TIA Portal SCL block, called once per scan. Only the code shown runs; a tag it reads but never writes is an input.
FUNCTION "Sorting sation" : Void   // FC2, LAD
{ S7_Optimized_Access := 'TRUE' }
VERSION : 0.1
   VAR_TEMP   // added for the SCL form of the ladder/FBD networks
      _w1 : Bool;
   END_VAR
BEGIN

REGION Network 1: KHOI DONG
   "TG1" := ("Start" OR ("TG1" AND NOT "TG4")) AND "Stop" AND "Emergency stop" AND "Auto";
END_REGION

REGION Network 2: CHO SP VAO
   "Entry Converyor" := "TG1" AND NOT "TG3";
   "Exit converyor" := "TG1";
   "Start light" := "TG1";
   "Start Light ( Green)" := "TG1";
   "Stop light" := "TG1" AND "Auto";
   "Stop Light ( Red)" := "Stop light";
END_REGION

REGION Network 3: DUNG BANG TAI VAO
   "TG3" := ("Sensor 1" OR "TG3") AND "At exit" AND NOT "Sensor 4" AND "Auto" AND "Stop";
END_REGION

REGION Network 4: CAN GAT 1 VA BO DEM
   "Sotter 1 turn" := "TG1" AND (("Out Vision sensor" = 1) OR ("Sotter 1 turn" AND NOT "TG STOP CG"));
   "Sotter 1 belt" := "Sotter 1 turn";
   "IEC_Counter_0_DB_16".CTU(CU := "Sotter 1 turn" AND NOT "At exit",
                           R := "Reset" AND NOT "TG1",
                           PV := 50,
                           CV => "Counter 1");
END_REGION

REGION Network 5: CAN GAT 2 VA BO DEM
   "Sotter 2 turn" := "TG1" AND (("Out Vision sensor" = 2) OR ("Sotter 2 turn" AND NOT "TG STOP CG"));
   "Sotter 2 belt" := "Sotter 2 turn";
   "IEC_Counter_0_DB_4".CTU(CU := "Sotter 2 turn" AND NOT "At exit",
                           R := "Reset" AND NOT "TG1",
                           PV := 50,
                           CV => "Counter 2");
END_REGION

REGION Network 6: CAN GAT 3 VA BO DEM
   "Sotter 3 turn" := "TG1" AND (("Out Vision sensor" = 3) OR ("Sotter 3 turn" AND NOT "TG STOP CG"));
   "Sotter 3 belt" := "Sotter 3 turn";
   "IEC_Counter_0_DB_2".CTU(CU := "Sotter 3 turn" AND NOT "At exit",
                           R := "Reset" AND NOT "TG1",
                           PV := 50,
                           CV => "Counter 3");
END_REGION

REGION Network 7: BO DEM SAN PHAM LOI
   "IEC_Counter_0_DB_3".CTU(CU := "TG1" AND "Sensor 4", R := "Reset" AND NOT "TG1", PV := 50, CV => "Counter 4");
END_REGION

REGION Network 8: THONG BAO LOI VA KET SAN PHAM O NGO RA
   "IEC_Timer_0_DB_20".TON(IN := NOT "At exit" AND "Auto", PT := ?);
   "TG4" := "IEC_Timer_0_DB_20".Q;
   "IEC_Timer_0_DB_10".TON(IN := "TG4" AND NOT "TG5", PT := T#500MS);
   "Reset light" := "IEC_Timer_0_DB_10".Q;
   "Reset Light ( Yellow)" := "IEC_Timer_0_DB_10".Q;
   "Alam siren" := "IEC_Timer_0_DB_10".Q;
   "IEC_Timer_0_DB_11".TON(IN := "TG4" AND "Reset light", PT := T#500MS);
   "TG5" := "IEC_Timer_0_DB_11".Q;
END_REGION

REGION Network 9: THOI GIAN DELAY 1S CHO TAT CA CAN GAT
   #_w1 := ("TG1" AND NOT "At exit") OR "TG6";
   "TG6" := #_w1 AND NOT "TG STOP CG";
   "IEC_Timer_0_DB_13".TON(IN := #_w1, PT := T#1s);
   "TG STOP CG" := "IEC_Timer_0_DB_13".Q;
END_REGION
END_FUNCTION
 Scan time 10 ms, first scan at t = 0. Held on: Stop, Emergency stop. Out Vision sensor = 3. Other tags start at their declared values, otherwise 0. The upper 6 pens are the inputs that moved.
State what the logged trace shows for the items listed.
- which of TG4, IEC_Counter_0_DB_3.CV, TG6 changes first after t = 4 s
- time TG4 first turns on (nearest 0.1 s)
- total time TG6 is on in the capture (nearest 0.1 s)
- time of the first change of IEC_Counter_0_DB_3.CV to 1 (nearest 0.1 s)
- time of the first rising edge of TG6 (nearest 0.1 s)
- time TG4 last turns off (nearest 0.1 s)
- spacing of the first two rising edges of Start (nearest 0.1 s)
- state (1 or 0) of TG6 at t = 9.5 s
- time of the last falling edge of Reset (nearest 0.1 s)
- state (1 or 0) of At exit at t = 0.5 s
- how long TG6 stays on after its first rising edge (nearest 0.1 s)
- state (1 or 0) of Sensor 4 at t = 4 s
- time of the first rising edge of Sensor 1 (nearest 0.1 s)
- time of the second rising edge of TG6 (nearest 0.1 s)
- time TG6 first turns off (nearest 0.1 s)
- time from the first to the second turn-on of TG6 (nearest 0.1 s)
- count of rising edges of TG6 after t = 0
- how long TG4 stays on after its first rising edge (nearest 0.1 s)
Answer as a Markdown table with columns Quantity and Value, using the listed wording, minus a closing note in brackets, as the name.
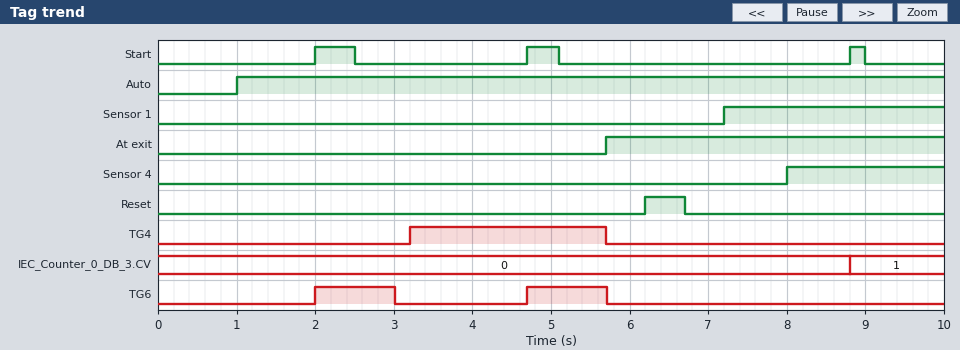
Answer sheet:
| Quantity | Value |
|---|---|
| which of TG4, IEC_Counter_0_DB_3.CV, TG6 changes first after t = 4 s | TG6 |
| time TG4 first turns on | 3.2 s |
| total time TG6 is on in the capture | 2.0 s |
| time of the first change of IEC_Counter_0_DB_3.CV to 1 | 8.8 s |
| time of the first rising edge of TG6 | 2.0 s |
| time TG4 last turns off | 5.7 s |
| spacing of the first two rising edges of Start | 2.7 s |
| state (1 or 0) of TG6 at t = 9.5 s | 0 |
| time of the last falling edge of Reset | 6.7 s |
| state (1 or 0) of At exit at t = 0.5 s | 0 |
| how long TG6 stays on after its first rising edge | 1.0 s |
| state (1 or 0) of Sensor 4 at t = 4 s | 0 |
| time of the first rising edge of Sensor 1 | 7.2 s |
| time of the second rising edge of TG6 | 4.7 s |
| time TG6 first turns off | 3.0 s |
| time from the first to the second turn-on of TG6 | 2.7 s |
| count of rising edges of TG6 after t = 0 | 2 |
| how long TG4 stays on after its first rising edge | 2.5 s |
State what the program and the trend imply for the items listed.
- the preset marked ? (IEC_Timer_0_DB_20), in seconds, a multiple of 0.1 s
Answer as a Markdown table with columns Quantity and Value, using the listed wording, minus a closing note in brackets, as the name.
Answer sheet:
| Quantity | Value |
|---|---|
| the preset marked ? (IEC_Timer_0_DB_20), in seconds, a multiple of 0.1 s | 2.2 s |
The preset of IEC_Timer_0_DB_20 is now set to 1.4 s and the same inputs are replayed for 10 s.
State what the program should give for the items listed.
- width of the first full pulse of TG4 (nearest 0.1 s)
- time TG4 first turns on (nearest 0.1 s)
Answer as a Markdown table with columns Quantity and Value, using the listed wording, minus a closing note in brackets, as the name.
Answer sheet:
| Quantity | Value |
|---|---|
| width of the first full pulse of TG4 | 3.3 s |
| time TG4 first turns on | 2.4 s |
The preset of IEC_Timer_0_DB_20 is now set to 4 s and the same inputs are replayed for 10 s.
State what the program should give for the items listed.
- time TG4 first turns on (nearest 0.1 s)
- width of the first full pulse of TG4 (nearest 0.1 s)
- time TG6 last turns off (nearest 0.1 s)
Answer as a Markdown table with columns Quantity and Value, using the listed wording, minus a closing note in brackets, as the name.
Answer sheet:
| Quantity | Value |
|---|---|
| time TG4 first turns on | 5.0 s |
| width of the first full pulse of TG4 | 0.7 s |
| time TG6 last turns off | 3.0 s |
